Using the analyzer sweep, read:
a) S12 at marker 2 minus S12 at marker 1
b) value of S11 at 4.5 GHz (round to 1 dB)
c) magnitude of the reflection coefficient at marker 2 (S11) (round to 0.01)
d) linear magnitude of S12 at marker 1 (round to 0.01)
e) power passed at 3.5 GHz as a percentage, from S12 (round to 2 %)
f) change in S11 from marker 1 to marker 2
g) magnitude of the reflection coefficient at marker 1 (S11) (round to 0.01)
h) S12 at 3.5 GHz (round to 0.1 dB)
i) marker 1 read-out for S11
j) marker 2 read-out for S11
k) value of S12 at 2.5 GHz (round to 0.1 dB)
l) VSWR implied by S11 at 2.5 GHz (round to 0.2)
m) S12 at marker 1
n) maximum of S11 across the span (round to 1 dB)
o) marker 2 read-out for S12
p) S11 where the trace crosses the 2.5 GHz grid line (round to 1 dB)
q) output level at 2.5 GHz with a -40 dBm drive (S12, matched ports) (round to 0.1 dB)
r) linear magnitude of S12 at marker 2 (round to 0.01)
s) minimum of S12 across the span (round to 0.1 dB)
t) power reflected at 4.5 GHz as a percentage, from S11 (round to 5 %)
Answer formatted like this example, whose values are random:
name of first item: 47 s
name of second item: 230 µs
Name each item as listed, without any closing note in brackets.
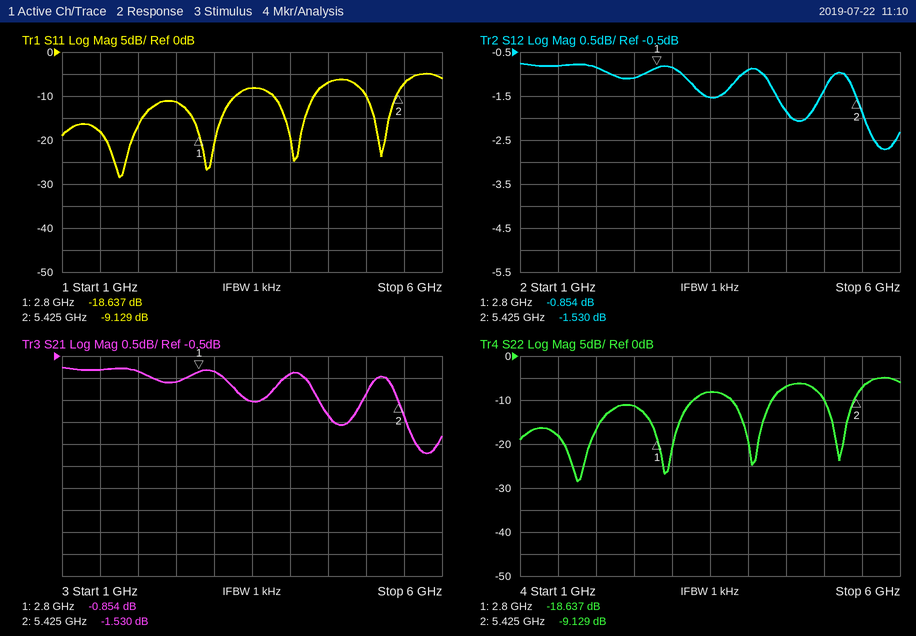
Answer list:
S12 at marker 2 minus S12 at marker 1: -0.676 dB
value of S11 at 4.5 GHz: -7 dB
magnitude of the reflection coefficient at marker 2 (S11): 0.35
linear magnitude of S12 at marker 1: 0.91
power passed at 3.5 GHz as a percentage, from S12: 70 %
change in S11 from marker 1 to marker 2: 9.508 dB
magnitude of the reflection coefficient at marker 1 (S11): 0.12
S12 at 3.5 GHz: -1.5 dB
marker 1 read-out for S11: -18.637 dB
marker 2 read-out for S11: -9.129 dB
value of S12 at 2.5 GHz: -1.1 dB
VSWR implied by S11 at 2.5 GHz: 1.8
S12 at marker 1: -0.854 dB
maximum of S11 across the span: -5 dB
marker 2 read-out for S12: -1.530 dB
S11 where the trace crosses the 2.5 GHz grid line: -11 dB
output level at 2.5 GHz with a -40 dBm drive (S12, matched ports): -41.1 dBm
linear magnitude of S12 at marker 2: 0.84
minimum of S12 across the span: -2.7 dB
power reflected at 4.5 GHz as a percentage, from S11: 20 %
